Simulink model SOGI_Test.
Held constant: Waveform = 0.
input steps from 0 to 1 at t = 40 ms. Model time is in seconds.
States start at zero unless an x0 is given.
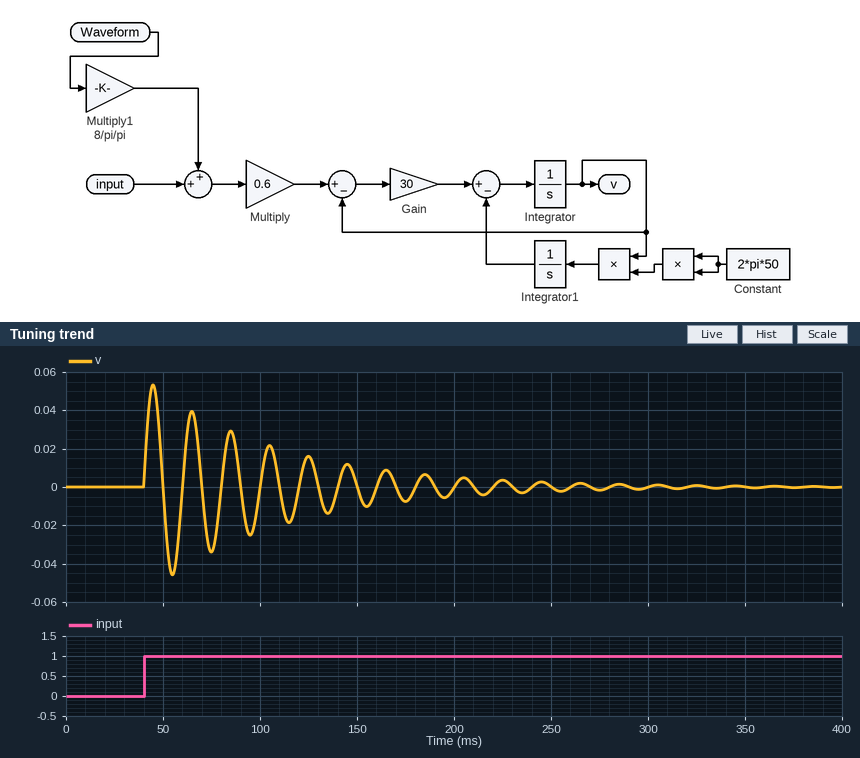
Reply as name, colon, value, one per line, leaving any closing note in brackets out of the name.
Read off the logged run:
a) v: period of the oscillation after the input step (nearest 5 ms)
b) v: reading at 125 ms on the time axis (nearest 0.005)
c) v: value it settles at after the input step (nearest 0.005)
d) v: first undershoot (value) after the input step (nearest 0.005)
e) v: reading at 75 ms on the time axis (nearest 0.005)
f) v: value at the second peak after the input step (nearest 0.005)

v: period of the oscillation after the input step: 20 ms
v: reading at 125 ms on the time axis: 0.015
v: value it settles at after the input step: 0.000
v: first undershoot (value) after the input step: -0.045
v: reading at 75 ms on the time axis: -0.035
v: value at the second peak after the input step: 0.040
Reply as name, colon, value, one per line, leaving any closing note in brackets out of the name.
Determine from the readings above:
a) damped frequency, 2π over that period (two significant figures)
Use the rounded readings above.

damped frequency, 2π over that period: 0.31 rad/ms
